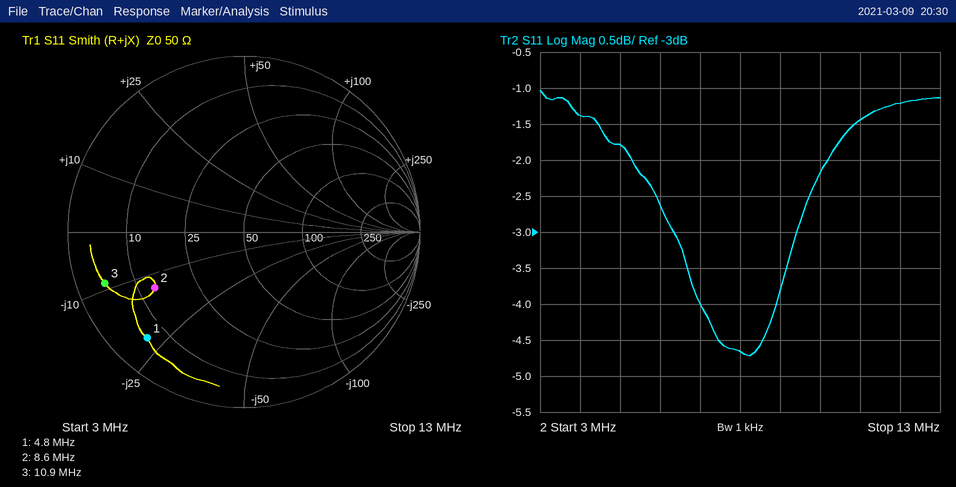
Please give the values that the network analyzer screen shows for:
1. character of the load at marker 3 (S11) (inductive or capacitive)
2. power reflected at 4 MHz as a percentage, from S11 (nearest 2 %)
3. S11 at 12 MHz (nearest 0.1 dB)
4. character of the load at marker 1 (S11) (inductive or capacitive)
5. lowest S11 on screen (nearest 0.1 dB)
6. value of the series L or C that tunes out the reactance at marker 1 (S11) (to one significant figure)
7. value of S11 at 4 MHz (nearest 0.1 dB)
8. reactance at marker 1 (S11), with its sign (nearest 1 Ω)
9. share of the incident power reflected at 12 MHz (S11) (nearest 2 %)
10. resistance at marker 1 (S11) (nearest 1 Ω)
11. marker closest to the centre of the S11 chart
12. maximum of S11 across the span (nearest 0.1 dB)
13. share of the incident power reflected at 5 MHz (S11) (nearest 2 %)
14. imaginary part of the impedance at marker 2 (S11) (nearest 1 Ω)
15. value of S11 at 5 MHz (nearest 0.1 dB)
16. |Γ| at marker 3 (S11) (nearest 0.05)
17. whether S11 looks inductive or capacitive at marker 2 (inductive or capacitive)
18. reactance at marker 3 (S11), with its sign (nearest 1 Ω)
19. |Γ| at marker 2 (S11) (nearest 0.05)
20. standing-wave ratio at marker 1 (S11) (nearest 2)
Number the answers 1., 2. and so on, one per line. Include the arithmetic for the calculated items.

1. capacitive
2. 10^(-1.4/10) ≈ 72 %
3. -1.2 dB
4. capacitive
5. -4.7 dB
6. L = 22 Ω/(2π × 4.8 MHz) ≈ 729 nH, so 700 nH to one significant figure
7. -1.4 dB
8. -22 Ω
9. 10^(-1.2/10) ≈ 76 %
10. 6 Ω
11. marker 2
12. -1.0 dB
13. 10^(-1.8/10) ≈ 66 %
14. -13 Ω
15. -1.8 dB
16. 0.85
17. capacitive
18. -9 Ω
19. 0.60
20. 10
